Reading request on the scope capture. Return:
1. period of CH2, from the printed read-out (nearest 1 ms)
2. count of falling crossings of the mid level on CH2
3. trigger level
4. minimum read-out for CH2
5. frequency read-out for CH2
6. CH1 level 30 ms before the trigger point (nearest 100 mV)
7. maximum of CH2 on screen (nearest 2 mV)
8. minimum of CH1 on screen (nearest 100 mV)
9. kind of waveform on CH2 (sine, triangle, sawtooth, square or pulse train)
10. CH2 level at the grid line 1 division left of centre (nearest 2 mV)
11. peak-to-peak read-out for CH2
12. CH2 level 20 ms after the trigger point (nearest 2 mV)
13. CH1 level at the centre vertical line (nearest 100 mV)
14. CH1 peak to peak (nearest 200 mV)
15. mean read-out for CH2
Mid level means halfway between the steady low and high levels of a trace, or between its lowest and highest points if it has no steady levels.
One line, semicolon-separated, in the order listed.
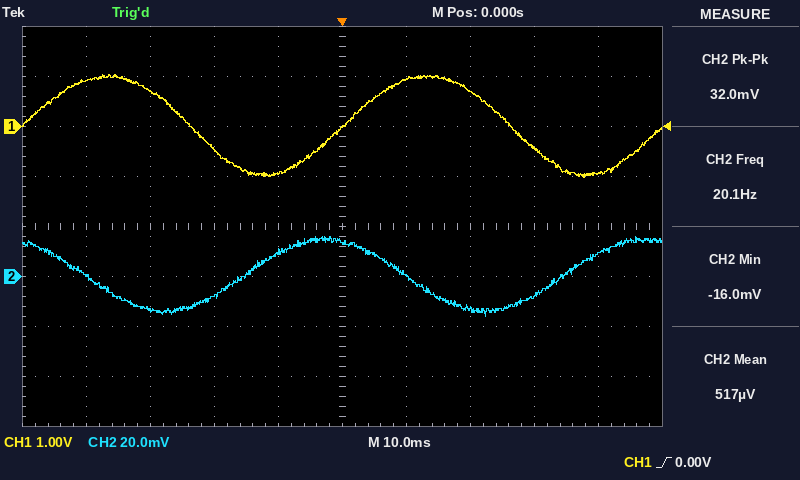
50 ms; 2; 0.00 V; -16.0 mV; 20.1 Hz; 700 mV; 16 mV; -1.0 V; sine; 10 mV; 32.0 mV; -14 mV; 0.0 V; 2.0 V; 517 µV
